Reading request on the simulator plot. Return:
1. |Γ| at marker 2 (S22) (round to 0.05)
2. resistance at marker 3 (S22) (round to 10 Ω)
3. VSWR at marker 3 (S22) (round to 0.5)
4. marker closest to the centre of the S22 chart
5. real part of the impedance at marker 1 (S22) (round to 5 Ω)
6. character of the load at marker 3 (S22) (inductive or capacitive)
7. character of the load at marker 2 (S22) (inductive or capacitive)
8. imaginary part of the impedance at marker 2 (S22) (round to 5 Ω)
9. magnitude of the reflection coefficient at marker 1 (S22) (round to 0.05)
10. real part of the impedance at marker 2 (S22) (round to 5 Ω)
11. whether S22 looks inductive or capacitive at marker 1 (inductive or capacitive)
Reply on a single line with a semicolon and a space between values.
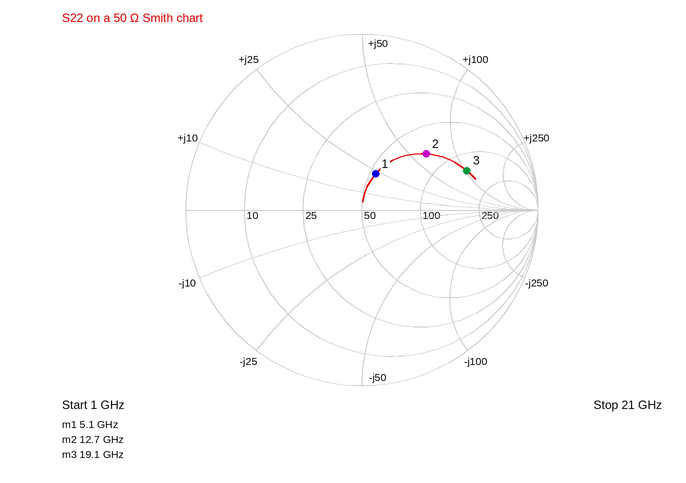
0.50; 140 Ω; 4.5; marker 1; 55 Ω; inductive; inductive; +65 Ω; 0.20; 75 Ω; inductive
